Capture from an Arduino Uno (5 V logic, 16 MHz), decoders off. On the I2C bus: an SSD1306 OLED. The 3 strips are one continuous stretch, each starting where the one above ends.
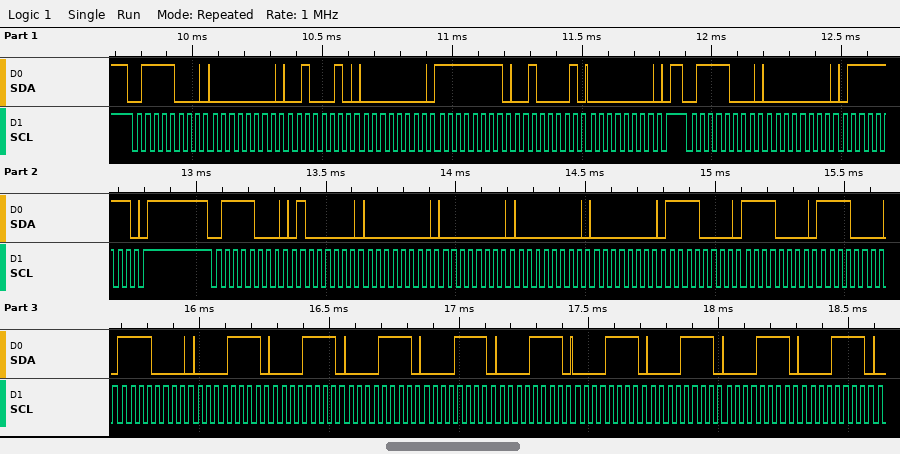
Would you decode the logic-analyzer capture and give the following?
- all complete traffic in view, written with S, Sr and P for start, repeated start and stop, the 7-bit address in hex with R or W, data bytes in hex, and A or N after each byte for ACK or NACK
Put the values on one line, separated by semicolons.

S 3CW A 00 A 22 A 00 A FF A 21 A 00 A P S 3CW A 00 A 7F A P S 3CW A 40 A 00 A 00 A 00 A 00 A F0 A F0 A F0 A F0 A 0F A 0F A 0F A 0F A 0F A 0F A 0F A 0F A 0F A
